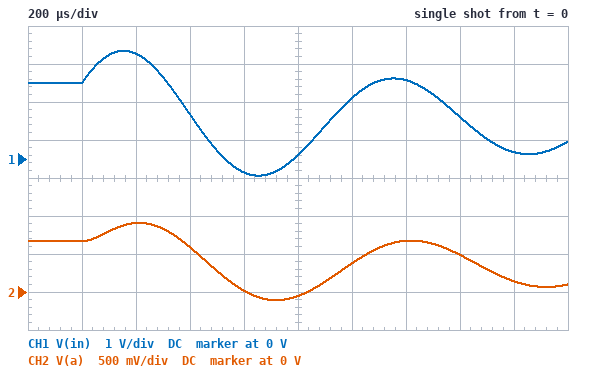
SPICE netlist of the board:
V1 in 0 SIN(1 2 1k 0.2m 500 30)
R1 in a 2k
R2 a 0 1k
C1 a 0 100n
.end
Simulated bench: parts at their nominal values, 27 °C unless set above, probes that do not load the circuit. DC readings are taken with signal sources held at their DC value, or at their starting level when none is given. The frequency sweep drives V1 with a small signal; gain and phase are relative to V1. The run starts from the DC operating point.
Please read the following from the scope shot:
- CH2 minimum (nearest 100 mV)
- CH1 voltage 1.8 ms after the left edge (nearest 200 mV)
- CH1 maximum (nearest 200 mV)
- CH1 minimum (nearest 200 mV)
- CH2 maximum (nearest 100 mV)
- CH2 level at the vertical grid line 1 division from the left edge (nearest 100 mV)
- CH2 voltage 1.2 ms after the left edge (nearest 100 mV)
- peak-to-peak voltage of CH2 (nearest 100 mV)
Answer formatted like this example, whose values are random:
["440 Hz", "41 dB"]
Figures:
["-100 mV", "200 mV", "2.8 V", "-400 mV", "900 mV", "700 mV", "400 mV", "1.0 V"]
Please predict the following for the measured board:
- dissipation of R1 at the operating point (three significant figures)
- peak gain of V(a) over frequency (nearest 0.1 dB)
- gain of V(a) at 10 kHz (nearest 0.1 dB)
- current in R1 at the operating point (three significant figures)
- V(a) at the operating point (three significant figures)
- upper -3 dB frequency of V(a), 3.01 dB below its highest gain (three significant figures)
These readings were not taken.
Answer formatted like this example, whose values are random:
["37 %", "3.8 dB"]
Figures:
["889 µW", "-9.5 dB", "-22.2 dB", "667 µA", "667 mV", "2.39 kHz"]
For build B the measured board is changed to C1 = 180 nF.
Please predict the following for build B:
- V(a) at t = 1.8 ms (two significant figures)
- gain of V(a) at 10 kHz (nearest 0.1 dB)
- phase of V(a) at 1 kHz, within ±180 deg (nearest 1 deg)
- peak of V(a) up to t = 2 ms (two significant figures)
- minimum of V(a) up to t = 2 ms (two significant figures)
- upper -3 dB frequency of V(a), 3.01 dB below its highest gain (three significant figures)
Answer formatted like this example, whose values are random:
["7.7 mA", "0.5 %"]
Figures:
["220 mV", "-27.2 dB", "-37 deg", "870 mV", "-43 mV", "1.33 kHz"]
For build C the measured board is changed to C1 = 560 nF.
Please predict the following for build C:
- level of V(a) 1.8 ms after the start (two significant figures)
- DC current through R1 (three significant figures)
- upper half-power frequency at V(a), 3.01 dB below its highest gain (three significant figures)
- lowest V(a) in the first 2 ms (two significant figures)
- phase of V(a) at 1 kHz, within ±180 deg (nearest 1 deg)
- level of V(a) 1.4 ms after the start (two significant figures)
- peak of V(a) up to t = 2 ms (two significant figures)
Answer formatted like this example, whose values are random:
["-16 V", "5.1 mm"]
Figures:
["350 mV", "667 µA", "426 Hz", "210 mV", "-67 deg", "430 mV", "780 mV"]
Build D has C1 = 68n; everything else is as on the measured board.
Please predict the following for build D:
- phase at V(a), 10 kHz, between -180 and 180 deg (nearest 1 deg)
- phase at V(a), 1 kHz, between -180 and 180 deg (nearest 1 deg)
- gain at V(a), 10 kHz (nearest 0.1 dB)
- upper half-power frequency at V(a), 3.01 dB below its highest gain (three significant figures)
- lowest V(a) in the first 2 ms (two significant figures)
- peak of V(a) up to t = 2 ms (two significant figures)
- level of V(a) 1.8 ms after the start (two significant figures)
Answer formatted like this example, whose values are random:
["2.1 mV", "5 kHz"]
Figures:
["-71 deg", "-16 deg", "-19.1 dB", "3.51 kHz", "-130 mV", "930 mV", "110 mV"]
